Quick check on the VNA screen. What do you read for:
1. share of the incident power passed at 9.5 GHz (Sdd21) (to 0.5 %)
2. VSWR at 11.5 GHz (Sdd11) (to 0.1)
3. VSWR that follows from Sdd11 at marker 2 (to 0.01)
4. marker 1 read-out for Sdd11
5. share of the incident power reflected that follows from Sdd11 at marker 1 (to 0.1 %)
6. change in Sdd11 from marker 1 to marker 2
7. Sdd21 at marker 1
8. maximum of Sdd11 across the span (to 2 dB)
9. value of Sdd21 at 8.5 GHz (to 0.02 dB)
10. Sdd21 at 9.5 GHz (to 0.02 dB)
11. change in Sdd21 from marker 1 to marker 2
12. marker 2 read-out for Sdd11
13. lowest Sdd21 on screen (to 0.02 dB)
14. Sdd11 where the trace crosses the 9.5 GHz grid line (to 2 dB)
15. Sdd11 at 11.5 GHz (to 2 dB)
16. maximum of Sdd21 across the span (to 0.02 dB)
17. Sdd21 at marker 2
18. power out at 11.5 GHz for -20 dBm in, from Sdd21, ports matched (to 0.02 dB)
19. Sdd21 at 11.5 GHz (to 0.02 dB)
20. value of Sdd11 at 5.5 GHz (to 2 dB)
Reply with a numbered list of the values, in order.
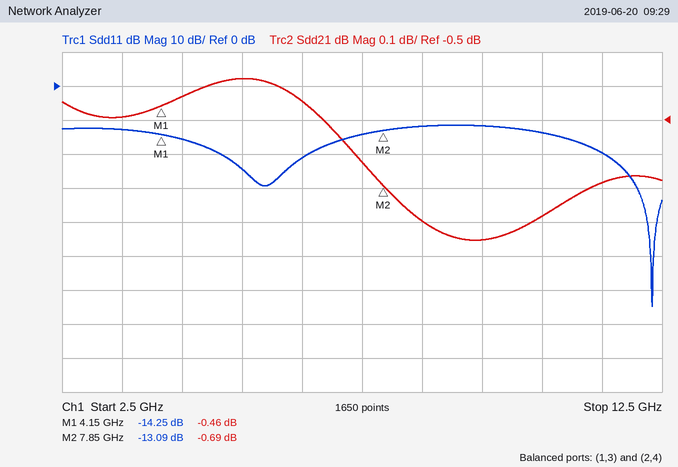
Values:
1. 82.0 %
2. 1.2
3. 1.57
4. -14.25 dB
5. 3.8 %
6. 1.16 dB
7. -0.46 dB
8. -12 dB
9. -0.80 dB
10. -0.86 dB
11. -0.23 dB
12. -13.09 dB
13. -0.86 dB
14. -12 dB
15. -20 dB
16. -0.38 dB
17. -0.69 dB
18. -20.68 dBm
19. -0.68 dB
20. -24 dB
